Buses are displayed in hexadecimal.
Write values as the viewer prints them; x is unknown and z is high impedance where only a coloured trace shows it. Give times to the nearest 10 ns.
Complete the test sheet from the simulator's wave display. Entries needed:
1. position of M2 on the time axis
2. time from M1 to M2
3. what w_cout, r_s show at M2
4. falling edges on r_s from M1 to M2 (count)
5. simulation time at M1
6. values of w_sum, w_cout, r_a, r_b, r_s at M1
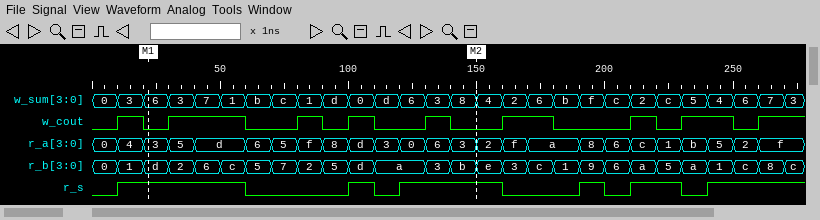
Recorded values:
150 ns
130 ns
w_cout=0, r_s=1
2
20 ns
w_sum=6, w_cout=0, r_a=3, r_b=d, r_s=1
